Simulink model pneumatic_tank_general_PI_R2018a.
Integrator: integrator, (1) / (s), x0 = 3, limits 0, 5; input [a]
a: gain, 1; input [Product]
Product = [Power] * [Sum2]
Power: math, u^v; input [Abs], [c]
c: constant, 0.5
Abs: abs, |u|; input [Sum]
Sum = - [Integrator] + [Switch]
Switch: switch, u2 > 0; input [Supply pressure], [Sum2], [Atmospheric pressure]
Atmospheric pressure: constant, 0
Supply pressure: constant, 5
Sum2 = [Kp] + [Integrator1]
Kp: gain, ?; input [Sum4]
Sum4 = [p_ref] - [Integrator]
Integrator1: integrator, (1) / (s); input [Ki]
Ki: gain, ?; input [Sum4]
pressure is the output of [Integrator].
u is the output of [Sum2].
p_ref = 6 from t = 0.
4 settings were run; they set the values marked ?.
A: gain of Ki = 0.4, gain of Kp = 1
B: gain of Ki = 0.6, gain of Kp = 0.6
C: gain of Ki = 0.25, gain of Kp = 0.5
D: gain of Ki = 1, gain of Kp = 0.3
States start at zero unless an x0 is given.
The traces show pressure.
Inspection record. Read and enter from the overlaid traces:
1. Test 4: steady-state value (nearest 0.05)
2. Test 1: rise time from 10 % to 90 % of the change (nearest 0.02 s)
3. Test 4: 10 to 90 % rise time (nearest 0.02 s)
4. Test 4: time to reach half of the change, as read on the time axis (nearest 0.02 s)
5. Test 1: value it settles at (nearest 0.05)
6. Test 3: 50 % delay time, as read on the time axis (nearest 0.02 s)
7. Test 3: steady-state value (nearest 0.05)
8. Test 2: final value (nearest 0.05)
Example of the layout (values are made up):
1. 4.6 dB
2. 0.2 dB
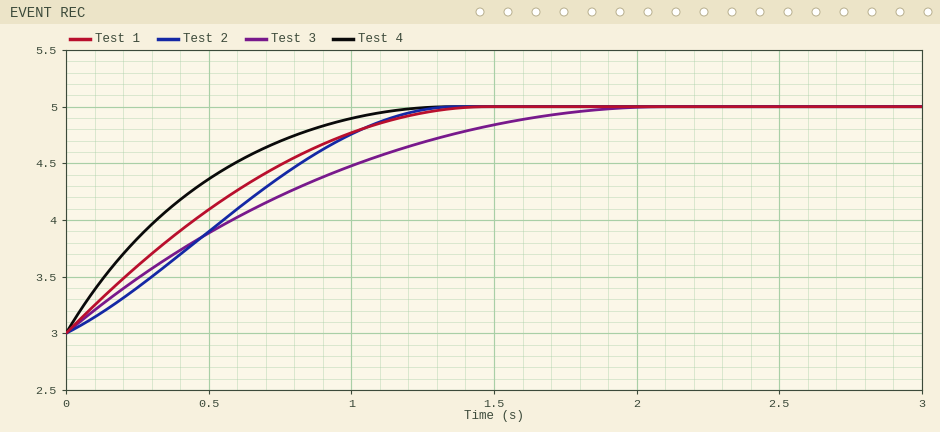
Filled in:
1. 5.00
2. 0.96 s
3. 0.82 s
4. 0.32 s
5. 5.00
6. 0.58 s
7. 5.00
8. 5.00
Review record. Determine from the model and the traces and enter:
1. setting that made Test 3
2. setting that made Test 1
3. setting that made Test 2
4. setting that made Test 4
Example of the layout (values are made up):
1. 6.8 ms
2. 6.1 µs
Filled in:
1. C
2. B
3. D
4. A
